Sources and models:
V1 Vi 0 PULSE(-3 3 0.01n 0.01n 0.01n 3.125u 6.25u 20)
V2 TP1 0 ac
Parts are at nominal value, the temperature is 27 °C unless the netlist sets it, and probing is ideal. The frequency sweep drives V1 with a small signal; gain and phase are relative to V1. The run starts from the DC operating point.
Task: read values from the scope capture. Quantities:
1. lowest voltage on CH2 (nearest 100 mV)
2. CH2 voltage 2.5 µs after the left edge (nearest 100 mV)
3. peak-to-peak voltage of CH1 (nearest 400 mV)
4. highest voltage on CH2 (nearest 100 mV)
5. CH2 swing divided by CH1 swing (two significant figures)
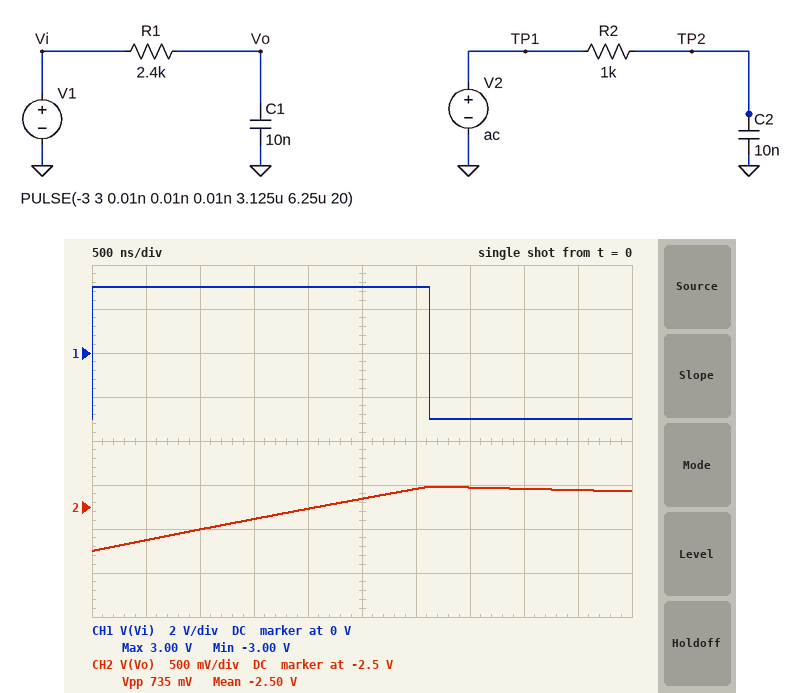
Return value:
-3.0 V
-2.4 V
6.0 V
-2.3 V
0.12
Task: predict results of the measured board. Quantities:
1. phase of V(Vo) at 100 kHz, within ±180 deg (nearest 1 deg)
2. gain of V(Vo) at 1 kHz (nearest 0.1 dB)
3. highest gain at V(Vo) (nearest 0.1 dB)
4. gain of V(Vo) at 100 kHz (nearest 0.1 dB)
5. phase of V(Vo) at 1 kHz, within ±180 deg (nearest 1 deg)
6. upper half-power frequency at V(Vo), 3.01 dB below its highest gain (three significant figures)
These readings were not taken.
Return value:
-86 deg
-0.1 dB
0 dB
-23.6 dB
-9 deg
6.63 kHz
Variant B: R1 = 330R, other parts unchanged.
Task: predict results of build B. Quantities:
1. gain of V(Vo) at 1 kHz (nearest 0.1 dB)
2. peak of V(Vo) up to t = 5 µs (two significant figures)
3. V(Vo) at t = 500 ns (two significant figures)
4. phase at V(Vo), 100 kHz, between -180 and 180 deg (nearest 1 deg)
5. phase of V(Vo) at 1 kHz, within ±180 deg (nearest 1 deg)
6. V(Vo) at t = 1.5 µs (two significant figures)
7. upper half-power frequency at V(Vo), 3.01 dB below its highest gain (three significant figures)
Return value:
0 dB
670 mV
-2.2 V
-64 deg
-1 deg
-810 mV
48.2 kHz
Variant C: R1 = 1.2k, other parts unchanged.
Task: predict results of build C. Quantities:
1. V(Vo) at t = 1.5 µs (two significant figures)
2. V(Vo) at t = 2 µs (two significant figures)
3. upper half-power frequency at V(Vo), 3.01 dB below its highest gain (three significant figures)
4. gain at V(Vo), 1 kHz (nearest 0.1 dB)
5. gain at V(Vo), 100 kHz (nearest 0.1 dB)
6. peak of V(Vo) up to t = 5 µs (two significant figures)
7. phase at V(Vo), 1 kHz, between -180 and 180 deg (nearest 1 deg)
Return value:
-2.3 V
-2.1 V
13.3 kHz
0 dB
-17.6 dB
-1.6 V
-4 deg
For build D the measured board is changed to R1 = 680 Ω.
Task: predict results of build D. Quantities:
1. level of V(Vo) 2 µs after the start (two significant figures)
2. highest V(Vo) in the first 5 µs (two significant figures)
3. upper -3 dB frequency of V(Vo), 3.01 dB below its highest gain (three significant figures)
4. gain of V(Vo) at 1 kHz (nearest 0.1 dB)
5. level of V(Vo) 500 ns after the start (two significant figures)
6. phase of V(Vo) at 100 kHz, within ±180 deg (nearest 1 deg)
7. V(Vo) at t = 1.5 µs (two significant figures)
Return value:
-1.5 V
-790 mV
23.4 kHz
0 dB
-2.6 V
-77 deg
-1.8 V
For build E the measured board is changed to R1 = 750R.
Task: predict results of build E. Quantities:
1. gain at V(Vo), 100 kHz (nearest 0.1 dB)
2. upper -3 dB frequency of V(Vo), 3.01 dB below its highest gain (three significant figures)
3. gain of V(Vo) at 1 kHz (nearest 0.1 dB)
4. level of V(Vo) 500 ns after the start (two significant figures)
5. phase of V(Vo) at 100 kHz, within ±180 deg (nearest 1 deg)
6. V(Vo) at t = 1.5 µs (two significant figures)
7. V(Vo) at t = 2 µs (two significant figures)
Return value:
-13.7 dB
21.2 kHz
0 dB
-2.6 V
-78 deg
-1.9 V
-1.6 V
